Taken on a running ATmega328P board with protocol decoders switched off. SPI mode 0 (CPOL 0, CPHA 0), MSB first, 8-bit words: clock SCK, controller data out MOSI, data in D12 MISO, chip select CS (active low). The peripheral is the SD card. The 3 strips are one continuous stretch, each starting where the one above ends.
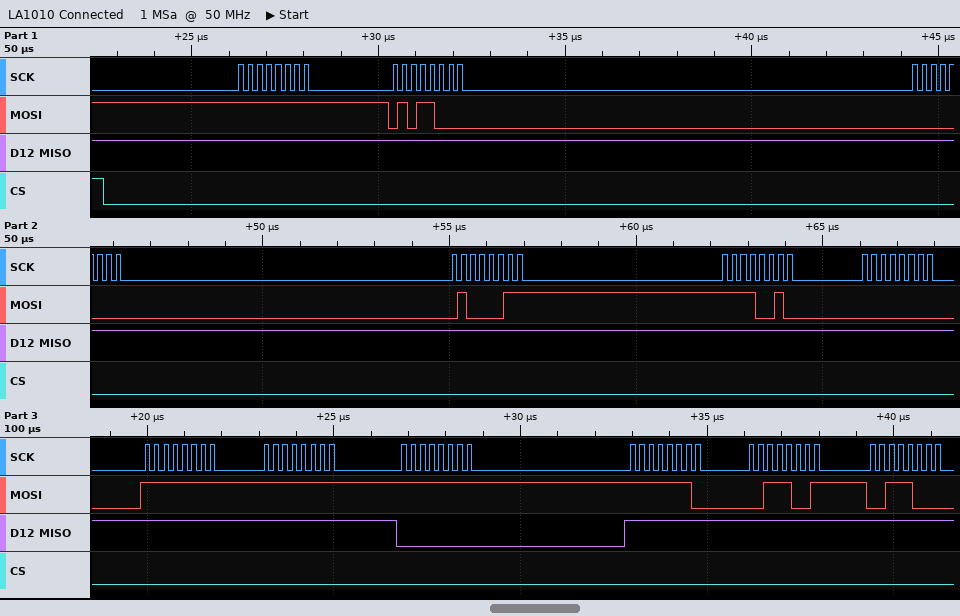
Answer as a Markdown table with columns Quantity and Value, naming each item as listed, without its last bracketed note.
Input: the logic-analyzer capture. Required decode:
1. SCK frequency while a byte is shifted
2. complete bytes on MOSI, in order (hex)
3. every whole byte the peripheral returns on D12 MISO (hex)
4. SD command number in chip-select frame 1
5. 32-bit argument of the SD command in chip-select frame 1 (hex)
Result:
| Quantity | Value |
|---|---|
| SCK frequency while a byte is shifted | 4 MHz |
| complete bytes on MOSI, in order | FF 58 00 43 F2 00 FF FF FF FE 39 38 |
| every whole byte the peripheral returns on D12 MISO | FF FF FF FF FF FF FF FF 00 FF FF FF |
| SD command number in chip-select frame 1 | CMD24 |
| 32-bit argument of the SD command in chip-select frame 1 | 0x0043F200 |
